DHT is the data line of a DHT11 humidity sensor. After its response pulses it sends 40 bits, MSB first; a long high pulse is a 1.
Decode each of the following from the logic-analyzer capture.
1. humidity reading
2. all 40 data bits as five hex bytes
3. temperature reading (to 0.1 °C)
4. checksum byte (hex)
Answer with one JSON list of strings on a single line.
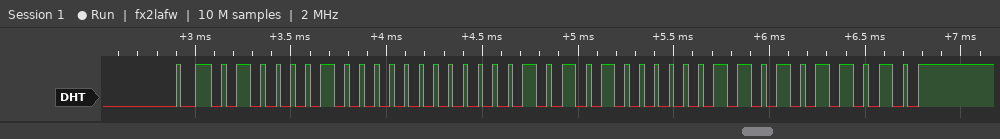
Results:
["66 %", "42 00 15 03 5A", "21.3 °C", "0x5A"]
